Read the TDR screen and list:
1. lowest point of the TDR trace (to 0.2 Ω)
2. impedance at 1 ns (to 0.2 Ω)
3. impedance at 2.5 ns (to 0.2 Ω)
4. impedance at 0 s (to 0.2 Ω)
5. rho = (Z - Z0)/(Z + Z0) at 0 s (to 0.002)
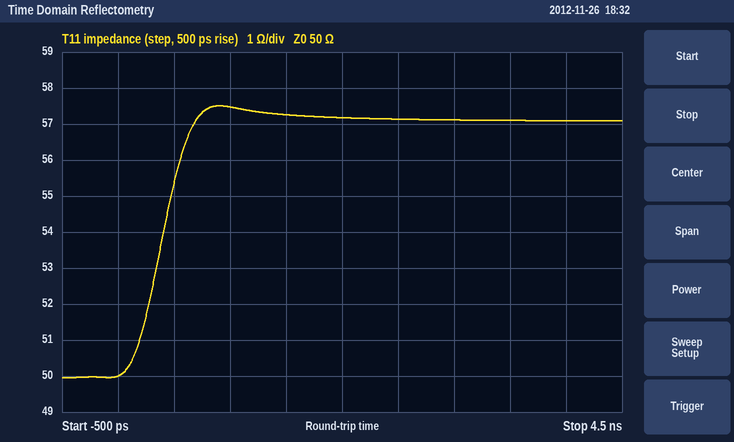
50.0 Ω
57.4 Ω
57.2 Ω
50.0 Ω
0.000
